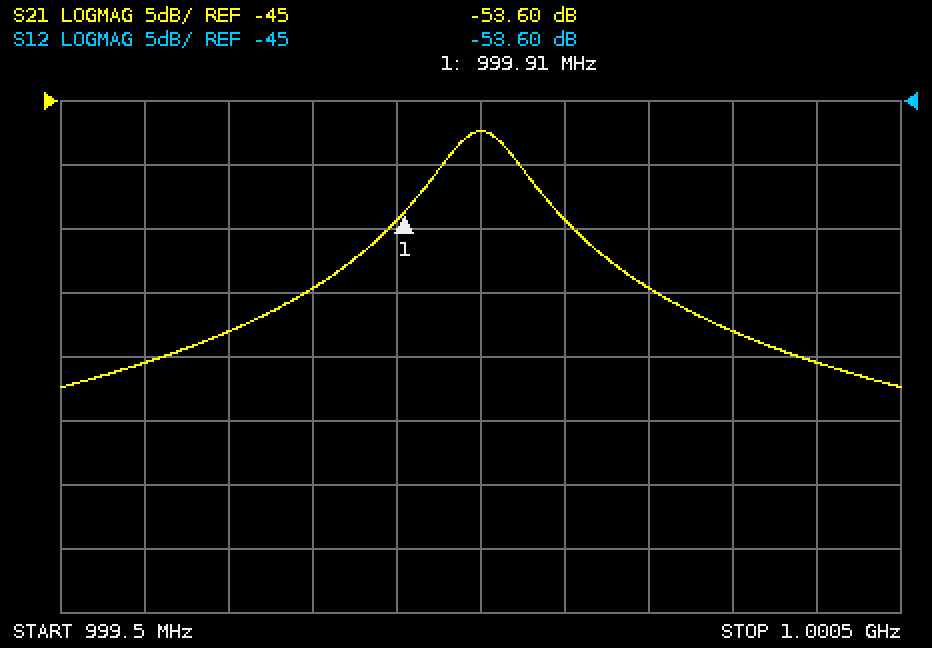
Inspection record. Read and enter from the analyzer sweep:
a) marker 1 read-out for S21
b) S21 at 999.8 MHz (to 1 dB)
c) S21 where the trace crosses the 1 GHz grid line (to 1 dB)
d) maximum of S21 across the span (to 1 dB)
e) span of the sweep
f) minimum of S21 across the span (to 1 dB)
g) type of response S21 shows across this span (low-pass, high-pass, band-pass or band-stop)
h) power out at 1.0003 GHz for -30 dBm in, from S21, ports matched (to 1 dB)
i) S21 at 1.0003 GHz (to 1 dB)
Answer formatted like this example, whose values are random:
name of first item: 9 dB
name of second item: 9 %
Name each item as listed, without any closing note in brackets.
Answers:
marker 1 read-out for S21: -53.60 dB
S21 at 999.8 MHz: -60 dB
S21 where the trace crosses the 1 GHz grid line: -47 dB
maximum of S21 across the span: -47 dB
span of the sweep: 1 MHz
minimum of S21 across the span: -67 dB
type of response S21 shows across this span: band-pass
power out at 1.0003 GHz for -30 dBm in, from S21, ports matched: -93 dBm
S21 at 1.0003 GHz: -63 dB
